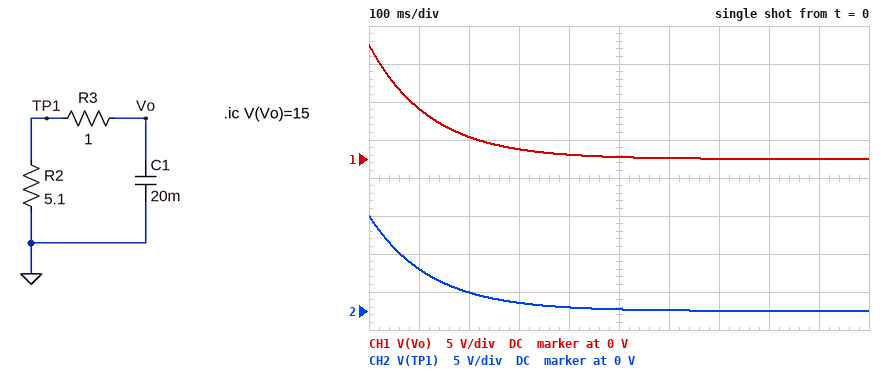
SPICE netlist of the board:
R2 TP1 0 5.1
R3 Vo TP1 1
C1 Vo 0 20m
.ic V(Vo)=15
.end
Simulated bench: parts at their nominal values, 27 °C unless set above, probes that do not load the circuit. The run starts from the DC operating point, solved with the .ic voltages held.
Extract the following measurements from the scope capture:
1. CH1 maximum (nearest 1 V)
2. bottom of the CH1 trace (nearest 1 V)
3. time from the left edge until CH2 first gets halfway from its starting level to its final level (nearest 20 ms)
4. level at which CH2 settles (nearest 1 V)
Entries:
15 V
0 V
80 ms
0 V
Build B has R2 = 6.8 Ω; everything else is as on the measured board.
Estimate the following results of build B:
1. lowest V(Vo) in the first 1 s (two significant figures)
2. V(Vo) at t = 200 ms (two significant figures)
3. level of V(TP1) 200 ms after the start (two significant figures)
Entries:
25 mV
4.2 V
3.6 V
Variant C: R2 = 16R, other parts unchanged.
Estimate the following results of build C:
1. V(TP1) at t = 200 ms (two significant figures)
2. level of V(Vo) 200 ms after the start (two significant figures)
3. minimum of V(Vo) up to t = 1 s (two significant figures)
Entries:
7.8 V
8.3 V
790 mV
